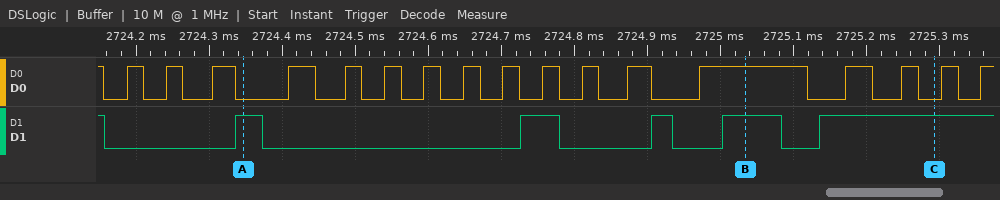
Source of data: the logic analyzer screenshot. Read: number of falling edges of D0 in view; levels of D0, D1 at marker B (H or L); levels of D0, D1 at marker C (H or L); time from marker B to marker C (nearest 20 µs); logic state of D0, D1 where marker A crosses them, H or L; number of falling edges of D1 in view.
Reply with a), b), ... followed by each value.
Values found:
a) 17
b) D0=H, D1=H
c) D0=L, D1=H
d) 260 µs
e) D0=L, D1=H
f) 5
